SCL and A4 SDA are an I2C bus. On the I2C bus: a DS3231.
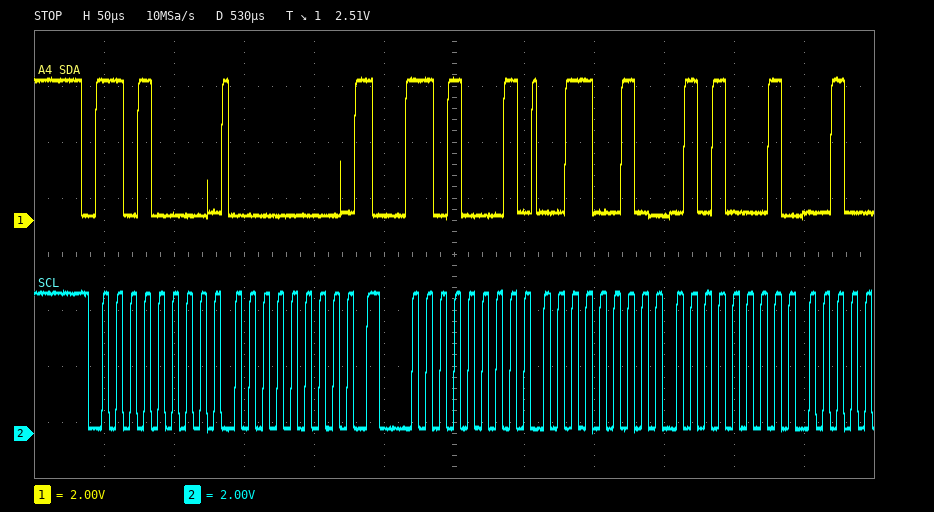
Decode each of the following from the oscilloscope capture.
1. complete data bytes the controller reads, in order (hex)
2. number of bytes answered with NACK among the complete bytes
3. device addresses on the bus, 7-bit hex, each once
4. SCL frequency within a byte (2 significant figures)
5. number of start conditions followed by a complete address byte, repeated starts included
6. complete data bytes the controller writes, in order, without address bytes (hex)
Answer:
32 51
0
0x68
100 kHz
2
00
